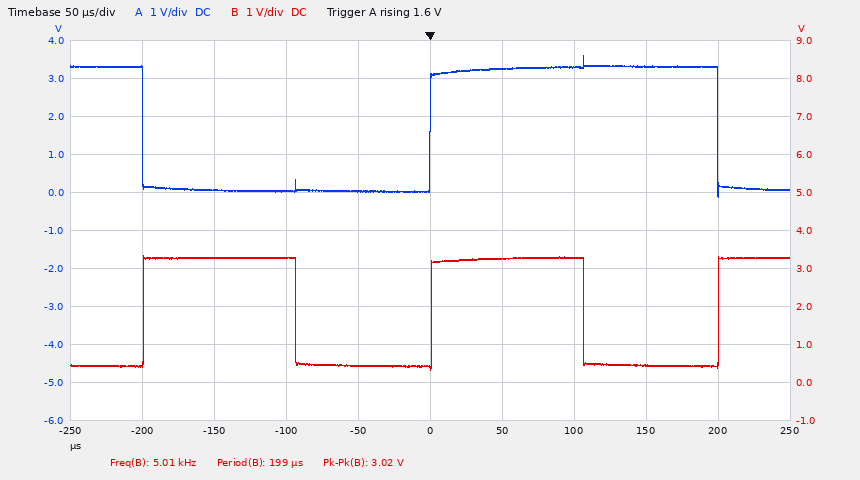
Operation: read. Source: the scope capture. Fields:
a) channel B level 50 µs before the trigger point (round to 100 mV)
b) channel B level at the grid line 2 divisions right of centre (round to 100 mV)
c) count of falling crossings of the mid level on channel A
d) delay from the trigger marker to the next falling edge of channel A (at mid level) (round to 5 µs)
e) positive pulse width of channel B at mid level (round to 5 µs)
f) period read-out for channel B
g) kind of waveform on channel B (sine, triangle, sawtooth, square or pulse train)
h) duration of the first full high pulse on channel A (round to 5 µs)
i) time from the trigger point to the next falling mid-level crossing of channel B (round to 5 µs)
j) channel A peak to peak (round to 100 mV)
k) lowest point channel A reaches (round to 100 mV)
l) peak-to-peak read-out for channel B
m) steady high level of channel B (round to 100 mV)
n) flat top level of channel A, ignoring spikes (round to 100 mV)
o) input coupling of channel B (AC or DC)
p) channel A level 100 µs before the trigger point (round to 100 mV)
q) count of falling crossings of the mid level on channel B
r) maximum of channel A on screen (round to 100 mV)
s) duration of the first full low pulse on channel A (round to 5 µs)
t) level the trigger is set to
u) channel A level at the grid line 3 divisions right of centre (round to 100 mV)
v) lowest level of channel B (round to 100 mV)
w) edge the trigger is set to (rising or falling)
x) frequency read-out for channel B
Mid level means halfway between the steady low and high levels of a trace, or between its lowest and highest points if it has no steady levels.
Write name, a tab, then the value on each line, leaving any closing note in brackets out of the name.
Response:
channel B level 50 µs before the trigger point	400 mV
channel B level at the grid line 2 divisions right of centre	3.3 V
count of falling crossings of the mid level on channel A	2
delay from the trigger marker to the next falling edge of channel A (at mid level)	200 µs
positive pulse width of channel B at mid level	105 µs
period read-out for channel B	199 µs
kind of waveform on channel B	square
duration of the first full high pulse on channel A	200 µs
time from the trigger point to the next falling mid-level crossing of channel B	105 µs
channel A peak to peak	3.7 V
lowest point channel A reaches	-100 mV
peak-to-peak read-out for channel B	3.02 V
steady high level of channel B	3.3 V
flat top level of channel A, ignoring spikes	3.3 V
input coupling of channel B	DC
channel A level 100 µs before the trigger point	0.0 V
count of falling crossings of the mid level on channel B	2
maximum of channel A on screen	3.6 V
duration of the first full low pulse on channel A	200 µs
level the trigger is set to	1.6 V
channel A level at the grid line 3 divisions right of centre	3.3 V
lowest level of channel B	300 mV
edge the trigger is set to	rising
frequency read-out for channel B	5.01 kHz
